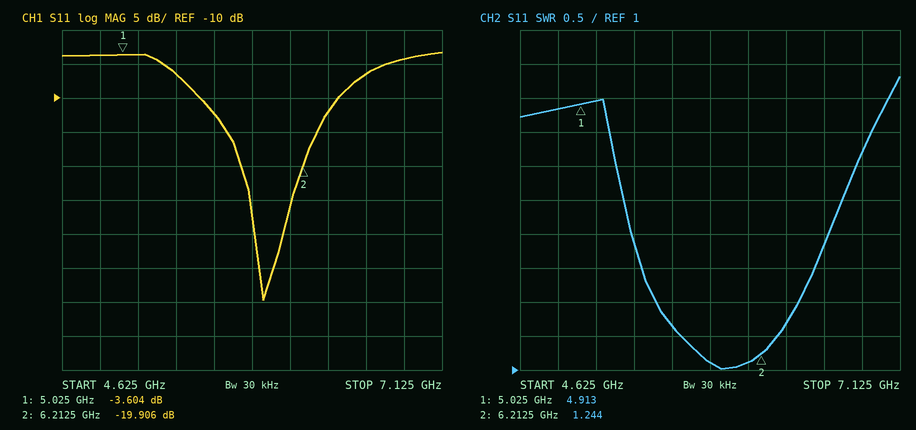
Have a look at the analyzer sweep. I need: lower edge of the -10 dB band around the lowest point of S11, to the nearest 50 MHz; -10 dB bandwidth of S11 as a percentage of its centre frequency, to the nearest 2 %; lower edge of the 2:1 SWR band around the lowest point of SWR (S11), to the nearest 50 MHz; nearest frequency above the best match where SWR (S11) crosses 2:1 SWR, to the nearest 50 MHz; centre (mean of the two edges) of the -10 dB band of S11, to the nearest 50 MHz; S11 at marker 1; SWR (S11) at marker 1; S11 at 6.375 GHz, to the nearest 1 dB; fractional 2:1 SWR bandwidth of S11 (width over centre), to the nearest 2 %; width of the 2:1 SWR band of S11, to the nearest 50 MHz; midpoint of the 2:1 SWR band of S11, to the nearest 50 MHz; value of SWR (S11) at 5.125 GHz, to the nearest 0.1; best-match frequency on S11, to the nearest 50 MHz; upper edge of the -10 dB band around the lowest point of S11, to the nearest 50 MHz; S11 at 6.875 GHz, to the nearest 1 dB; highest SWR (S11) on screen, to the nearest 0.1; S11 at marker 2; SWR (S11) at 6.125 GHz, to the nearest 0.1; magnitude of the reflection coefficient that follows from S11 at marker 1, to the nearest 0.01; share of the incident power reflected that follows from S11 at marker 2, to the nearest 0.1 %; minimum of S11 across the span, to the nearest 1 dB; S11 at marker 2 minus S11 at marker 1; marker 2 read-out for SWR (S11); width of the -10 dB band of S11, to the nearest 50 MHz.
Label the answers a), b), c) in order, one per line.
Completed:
a) 5.55 GHz
b) 16 %
c) 5.50 GHz
d) 6.45 GHz
e) 6.00 GHz
f) -3.604 dB
g) 4.913
h) -12 dB
i) 16 %
j) 950 MHz
k) 6.00 GHz
l) 5.0
m) 5.95 GHz
n) 6.45 GHz
o) -4 dB
p) 5.3
q) -19.906 dB
r) 1.1
s) 0.66
t) 1.0 %
u) -40 dB
v) -16.302 dB
w) 1.244
x) 900 MHz
